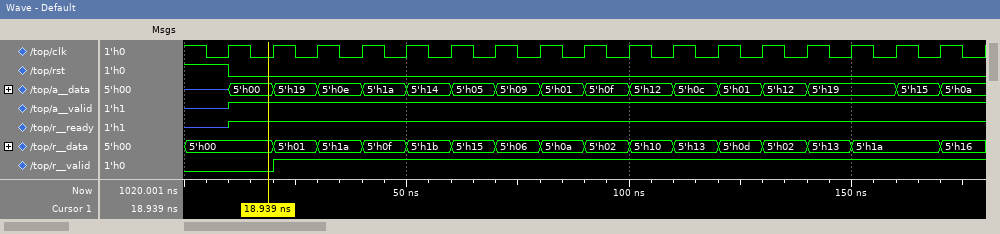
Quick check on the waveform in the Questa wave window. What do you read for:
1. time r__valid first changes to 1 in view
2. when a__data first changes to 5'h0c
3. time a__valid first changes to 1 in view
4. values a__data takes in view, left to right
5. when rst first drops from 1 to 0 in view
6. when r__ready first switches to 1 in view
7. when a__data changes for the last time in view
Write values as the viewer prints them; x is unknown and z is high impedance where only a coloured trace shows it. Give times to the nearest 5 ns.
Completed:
20 ns
110 ns
10 ns
z, 5'h00, 5'h19, 5'h0e, 5'h1a, 5'h14, 5'h05, 5'h09, 5'h01, 5'h0f, 5'h12, 5'h0c, 5'h01, 5'h12, 5'h19, 5'h15, 5'h0a
10 ns
10 ns
170 ns
